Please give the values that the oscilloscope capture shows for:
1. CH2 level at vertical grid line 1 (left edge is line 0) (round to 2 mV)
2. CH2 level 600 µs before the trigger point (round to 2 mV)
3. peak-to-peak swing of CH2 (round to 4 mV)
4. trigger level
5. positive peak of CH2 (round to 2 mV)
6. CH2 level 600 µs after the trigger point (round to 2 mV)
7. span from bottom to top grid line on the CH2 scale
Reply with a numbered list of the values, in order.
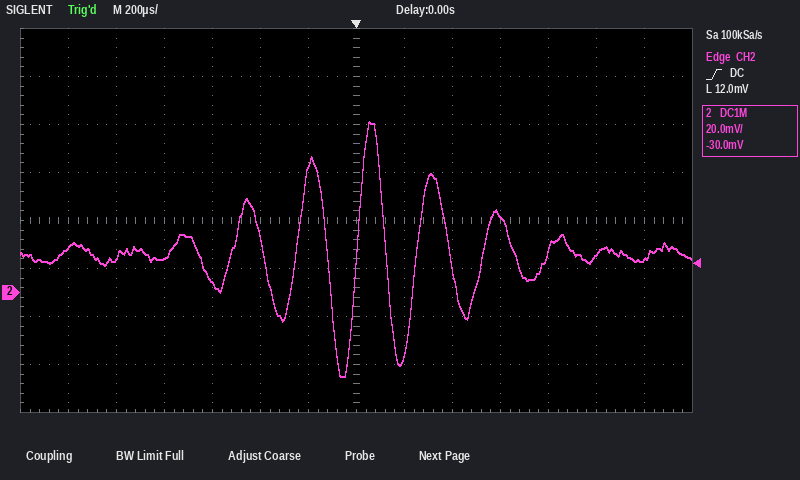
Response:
1. 18 mV
2. 4 mV
3. 108 mV
4. 12.0 mV
5. 72 mV
6. 32 mV
7. 160 mV
